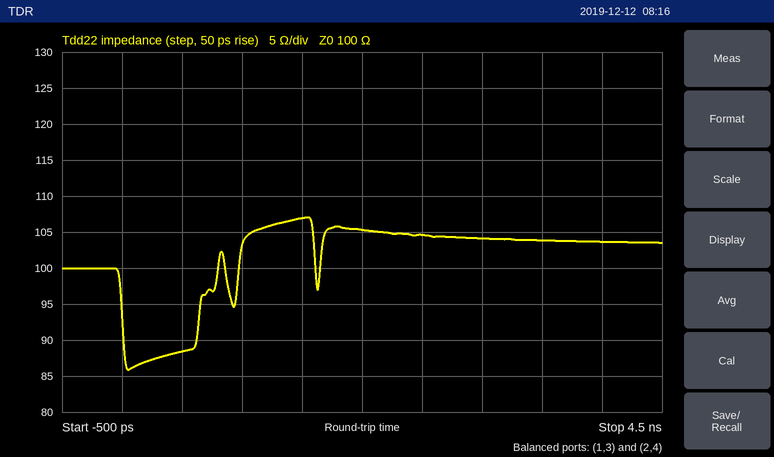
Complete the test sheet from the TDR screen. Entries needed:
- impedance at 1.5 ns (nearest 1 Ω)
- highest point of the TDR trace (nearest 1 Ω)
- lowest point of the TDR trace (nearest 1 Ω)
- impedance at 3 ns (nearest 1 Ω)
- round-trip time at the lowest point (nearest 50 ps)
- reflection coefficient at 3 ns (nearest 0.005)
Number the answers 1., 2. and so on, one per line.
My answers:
1. 107 Ω
2. 107 Ω
3. 86 Ω
4. 104 Ω
5. 50 ps
6. +0.020
